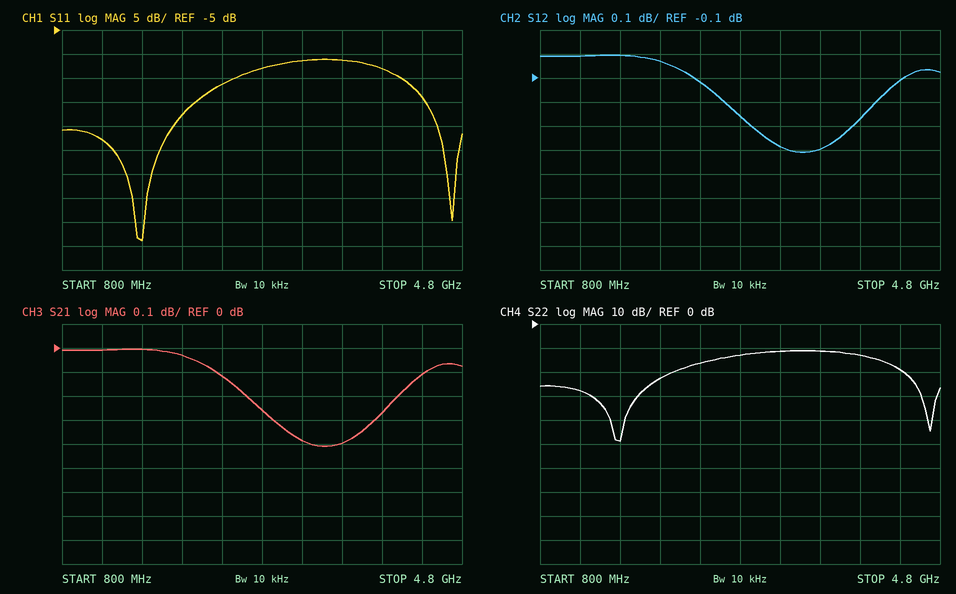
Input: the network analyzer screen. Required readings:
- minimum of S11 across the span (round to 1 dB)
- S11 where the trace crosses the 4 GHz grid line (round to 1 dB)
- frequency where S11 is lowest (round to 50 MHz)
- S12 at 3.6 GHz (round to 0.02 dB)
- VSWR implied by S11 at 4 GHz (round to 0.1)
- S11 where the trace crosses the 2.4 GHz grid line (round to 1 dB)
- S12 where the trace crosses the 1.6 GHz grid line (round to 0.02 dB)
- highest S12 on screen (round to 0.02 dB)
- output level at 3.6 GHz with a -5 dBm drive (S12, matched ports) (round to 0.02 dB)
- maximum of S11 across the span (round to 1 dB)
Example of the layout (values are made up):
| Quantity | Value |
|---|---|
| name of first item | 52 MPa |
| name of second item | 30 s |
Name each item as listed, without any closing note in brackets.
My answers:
| Quantity | Value |
|---|---|
| minimum of S11 across the span | -49 dB |
| S11 where the trace crosses the 4 GHz grid line | -13 dB |
| frequency where S11 is lowest | 1.60 GHz |
| S12 at 3.6 GHz | -0.40 dB |
| VSWR implied by S11 at 4 GHz | 1.6 |
| S11 where the trace crosses the 2.4 GHz grid line | -16 dB |
| S12 where the trace crosses the 1.6 GHz grid line | 0.00 dB |
| highest S12 on screen | 0.00 dB |
| output level at 3.6 GHz with a -5 dBm drive (S12, matched ports) | -5.40 dBm |
| maximum of S11 across the span | -11 dB |
